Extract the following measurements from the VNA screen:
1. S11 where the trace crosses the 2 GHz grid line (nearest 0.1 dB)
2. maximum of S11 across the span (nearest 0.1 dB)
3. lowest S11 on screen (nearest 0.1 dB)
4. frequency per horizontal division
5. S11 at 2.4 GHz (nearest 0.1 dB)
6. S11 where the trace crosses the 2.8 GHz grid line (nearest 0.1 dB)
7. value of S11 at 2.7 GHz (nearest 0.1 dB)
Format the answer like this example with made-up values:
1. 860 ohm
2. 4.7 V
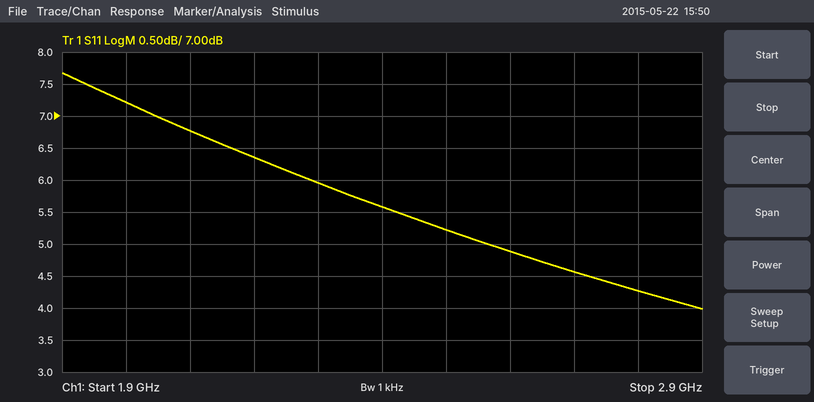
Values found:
1. 7.2 dB
2. 7.7 dB
3. 4.0 dB
4. 100 MHz
5. 5.6 dB
6. 4.3 dB
7. 4.6 dB
